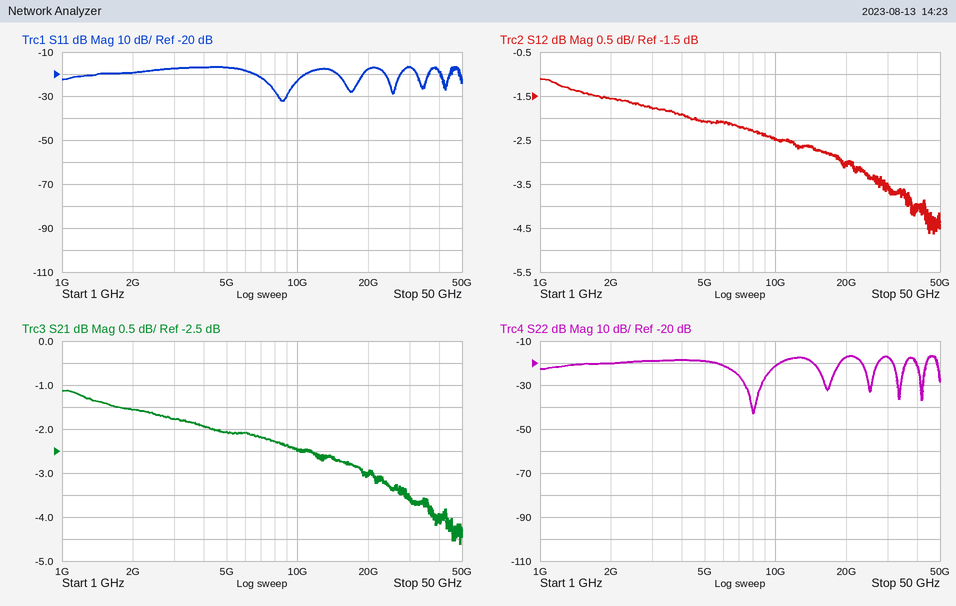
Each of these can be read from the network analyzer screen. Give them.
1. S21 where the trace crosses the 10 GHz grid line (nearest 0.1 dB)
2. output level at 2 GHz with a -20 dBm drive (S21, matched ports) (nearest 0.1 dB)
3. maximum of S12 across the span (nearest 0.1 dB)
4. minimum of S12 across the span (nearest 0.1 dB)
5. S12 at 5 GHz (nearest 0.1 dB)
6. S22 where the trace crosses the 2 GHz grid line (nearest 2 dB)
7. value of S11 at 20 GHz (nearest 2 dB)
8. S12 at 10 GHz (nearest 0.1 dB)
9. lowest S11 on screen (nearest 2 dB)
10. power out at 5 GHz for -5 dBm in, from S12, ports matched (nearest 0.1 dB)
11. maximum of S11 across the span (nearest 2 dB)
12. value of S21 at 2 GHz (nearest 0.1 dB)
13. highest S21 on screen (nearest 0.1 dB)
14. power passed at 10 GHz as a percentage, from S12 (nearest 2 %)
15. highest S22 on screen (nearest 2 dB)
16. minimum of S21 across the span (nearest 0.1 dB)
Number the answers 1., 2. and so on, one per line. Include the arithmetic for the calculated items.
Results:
1. -2.5 dB
2. -20 dBm + (-1.6 dB) = -21.6 dBm
3. -1.1 dB
4. -4.6 dB
5. -2.1 dB
6. -20 dB
7. -18 dB
8. -2.5 dB
9. -32 dB
10. -5 dBm + (-2.1 dB) = -7.1 dBm
11. -16 dB
12. -1.6 dB
13. -1.1 dB
14. 10^(-2.5/10) ≈ 56 %
15. -16 dB
16. -4.6 dB
